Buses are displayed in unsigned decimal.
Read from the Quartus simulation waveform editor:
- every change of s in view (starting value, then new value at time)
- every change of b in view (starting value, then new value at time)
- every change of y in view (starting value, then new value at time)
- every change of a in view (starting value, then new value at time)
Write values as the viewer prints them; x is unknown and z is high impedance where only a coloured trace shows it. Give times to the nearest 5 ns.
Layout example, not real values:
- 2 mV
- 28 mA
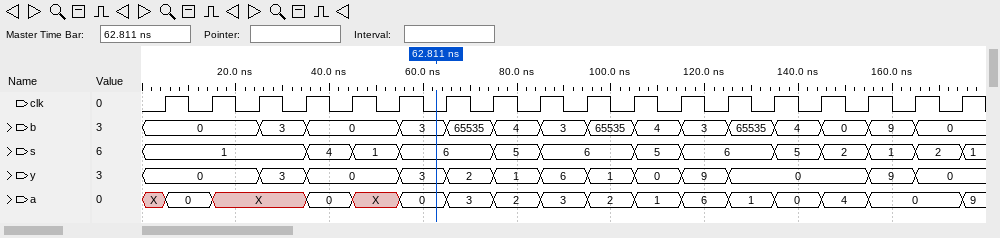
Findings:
- 1, 4 at 35 ns, 1 at 45 ns, 6 at 55 ns, 5 at 75 ns, 6 at 85 ns, 5 at 105 ns, 6 at 115 ns, 5 at 135 ns, 2 at 145 ns, 1 at 155 ns, 2 at 165 ns, 1 at 175 ns
- 0, 3 at 25 ns, 0 at 35 ns, 3 at 55 ns, 65535 at 65 ns, 4 at 75 ns, 3 at 85 ns, 65535 at 95 ns, 4 at 105 ns, 3 at 115 ns, 65535 at 125 ns, 4 at 135 ns, 0 at 145 ns, 9 at 155 ns, 0 at 165 ns
- 0, 3 at 25 ns, 0 at 35 ns, 3 at 55 ns, 2 at 65 ns, 1 at 75 ns, 6 at 85 ns, 1 at 95 ns, 0 at 105 ns, 9 at 115 ns, 0 at 125 ns, 9 at 155 ns, 0 at 165 ns
- X, 0 at 5 ns, X at 15 ns, 0 at 35 ns, X at 45 ns, 0 at 55 ns, 3 at 65 ns, 2 at 75 ns, 3 at 85 ns, 2 at 95 ns, 1 at 105 ns, 6 at 115 ns, 1 at 125 ns, 0 at 135 ns, 4 at 145 ns, 0 at 155 ns, 9 at 175 ns
